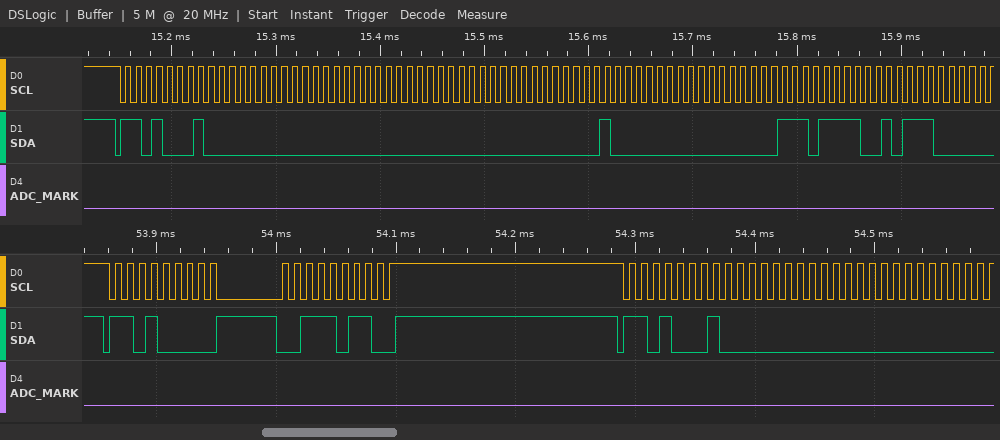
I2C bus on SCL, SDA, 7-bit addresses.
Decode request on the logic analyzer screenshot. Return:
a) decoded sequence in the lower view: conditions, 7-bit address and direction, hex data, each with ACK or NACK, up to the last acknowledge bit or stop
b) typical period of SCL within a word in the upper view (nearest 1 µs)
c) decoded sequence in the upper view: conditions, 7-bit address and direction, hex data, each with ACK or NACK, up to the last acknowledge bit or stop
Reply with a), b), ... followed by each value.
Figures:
a) start, address 68 write ACK, 3B ACK, stop, start, address 68 read ACK, 00 ACK, 00 ACK
b) 10 µs
c) start, address 68 read ACK, 00 ACK, 00 ACK, 00 ACK, 00 ACK, 40 ACK, 00 ACK, EF ACK, 5C ACK
